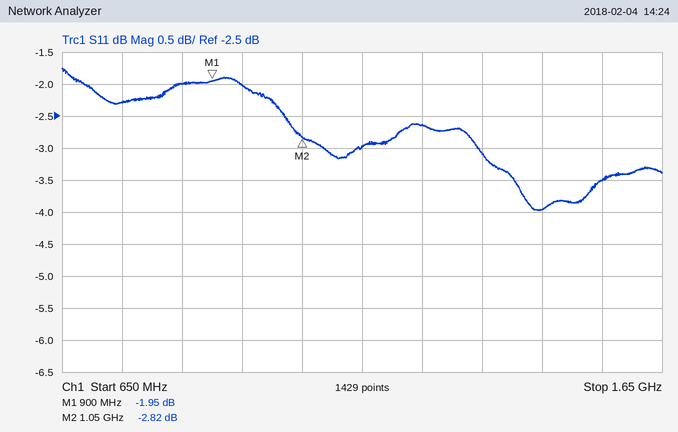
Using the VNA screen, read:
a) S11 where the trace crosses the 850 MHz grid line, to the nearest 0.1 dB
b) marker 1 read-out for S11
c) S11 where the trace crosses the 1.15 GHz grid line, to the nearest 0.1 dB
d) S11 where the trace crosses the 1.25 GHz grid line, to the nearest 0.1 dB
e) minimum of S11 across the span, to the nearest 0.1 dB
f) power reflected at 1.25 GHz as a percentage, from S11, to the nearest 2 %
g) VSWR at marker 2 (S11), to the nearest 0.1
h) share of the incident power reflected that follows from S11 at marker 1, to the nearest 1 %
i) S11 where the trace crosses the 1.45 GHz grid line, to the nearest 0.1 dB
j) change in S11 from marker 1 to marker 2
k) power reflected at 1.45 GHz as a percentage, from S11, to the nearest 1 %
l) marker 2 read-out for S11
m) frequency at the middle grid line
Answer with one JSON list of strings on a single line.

["-2.0 dB", "-1.95 dB", "-3.0 dB", "-2.6 dB", "-4.0 dB", "54 %", "6.2", "64 %", "-4.0 dB", "-0.87 dB", "40 %", "-2.82 dB", "1.15 GHz"]
